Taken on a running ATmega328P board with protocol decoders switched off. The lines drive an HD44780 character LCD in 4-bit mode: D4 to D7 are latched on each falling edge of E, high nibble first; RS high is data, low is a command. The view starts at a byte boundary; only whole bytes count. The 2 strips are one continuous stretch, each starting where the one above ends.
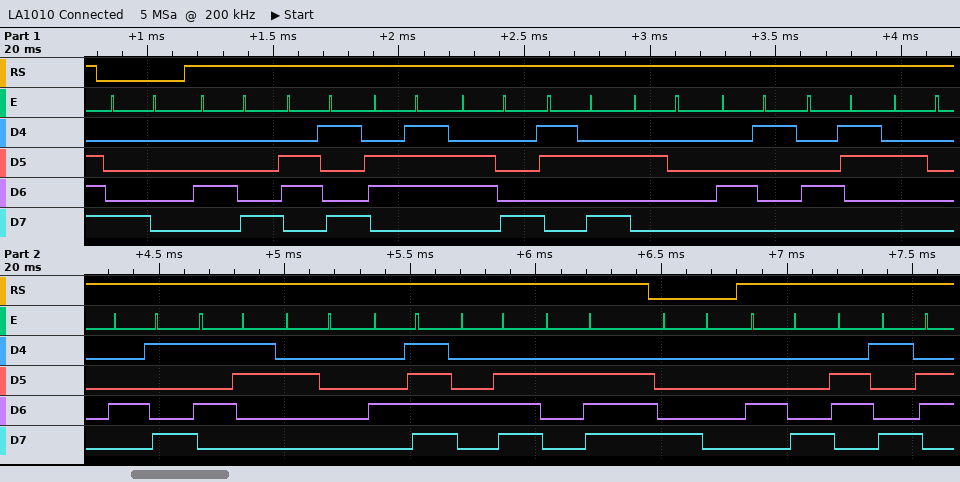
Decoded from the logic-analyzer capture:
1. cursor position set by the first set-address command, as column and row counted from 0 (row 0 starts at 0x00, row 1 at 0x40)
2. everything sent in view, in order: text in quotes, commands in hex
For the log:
column 0, row 0
0x80 "High: AC IS ON." 0x80 "Hi"
